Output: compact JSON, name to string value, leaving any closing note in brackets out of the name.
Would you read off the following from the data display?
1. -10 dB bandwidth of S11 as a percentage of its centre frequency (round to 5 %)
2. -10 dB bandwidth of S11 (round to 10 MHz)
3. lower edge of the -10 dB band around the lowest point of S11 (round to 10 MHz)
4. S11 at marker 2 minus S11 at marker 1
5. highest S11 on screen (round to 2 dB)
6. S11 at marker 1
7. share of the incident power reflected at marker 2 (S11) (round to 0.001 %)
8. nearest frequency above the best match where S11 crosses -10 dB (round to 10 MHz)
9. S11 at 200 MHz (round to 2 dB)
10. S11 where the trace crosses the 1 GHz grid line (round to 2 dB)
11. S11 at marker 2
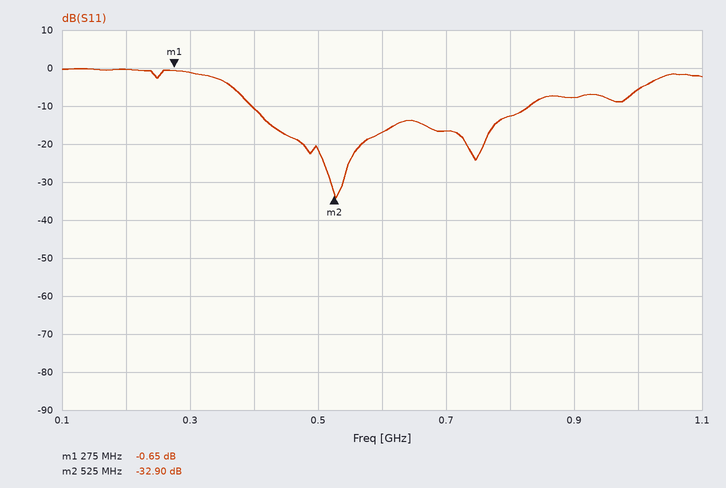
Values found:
{"-10 dB bandwidth of S11 as a percentage of its centre frequency": "70 %", "-10 dB bandwidth of S11": "430 MHz", "lower edge of the -10 dB band around the lowest point of S11": "400 MHz", "S11 at marker 2 minus S11 at marker 1": "-32.25 dB", "highest S11 on screen": "0 dB", "S11 at marker 1": "-0.65 dB", "share of the incident power reflected at marker 2 (S11)": "0.051 %", "nearest frequency above the best match where S11 crosses -10 dB": "830 MHz", "S11 at 200 MHz": "0 dB", "S11 where the trace crosses the 1 GHz grid line": "-6 dB", "S11 at marker 2": "-32.90 dB"}
